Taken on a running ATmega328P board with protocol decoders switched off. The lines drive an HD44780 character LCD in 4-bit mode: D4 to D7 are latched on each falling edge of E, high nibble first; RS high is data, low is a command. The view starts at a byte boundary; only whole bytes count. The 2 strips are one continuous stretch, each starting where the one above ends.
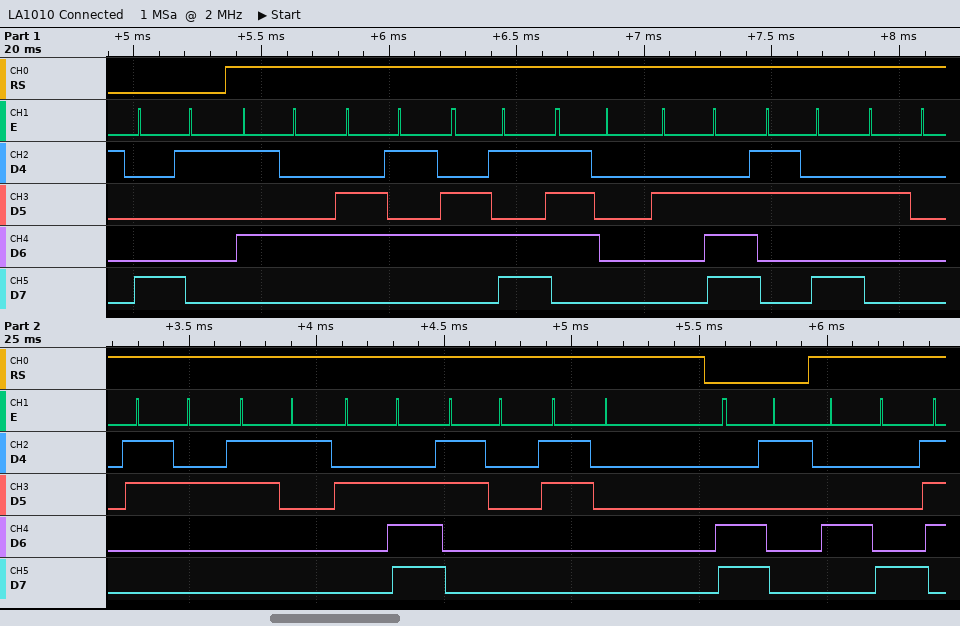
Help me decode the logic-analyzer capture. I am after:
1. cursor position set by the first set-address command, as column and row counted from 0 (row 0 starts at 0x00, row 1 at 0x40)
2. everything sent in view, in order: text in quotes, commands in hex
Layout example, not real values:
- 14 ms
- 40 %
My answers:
- column 1, row 0
- 0x81 "Temp.: 21.00" 0xC1 "H"
